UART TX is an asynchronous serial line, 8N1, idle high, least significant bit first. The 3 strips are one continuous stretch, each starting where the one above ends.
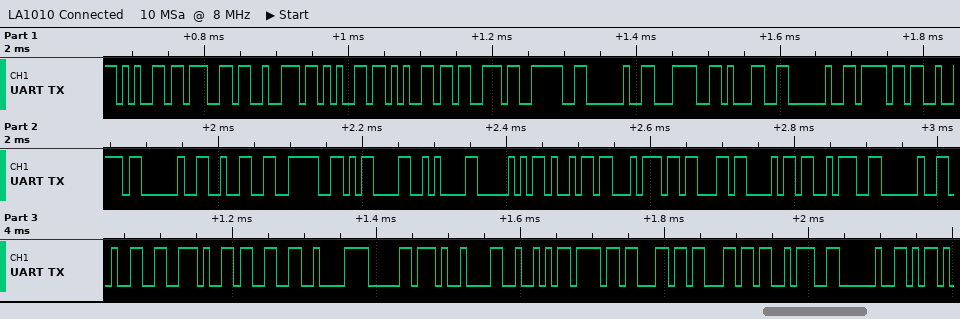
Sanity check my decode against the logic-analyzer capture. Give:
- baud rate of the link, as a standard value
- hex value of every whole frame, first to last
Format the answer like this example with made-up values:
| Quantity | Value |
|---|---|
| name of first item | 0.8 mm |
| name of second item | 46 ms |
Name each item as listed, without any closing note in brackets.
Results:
| Quantity | Value |
|---|---|
| baud rate of the link, as a standard value | 115200 baud |
| hex value of every whole frame, first to last | 65 67 72 65 65 73 3E 20 3C 31 20 6F 72 20 32 3E 0D 0A 50 69 74 63 68 3A 20 32 2E 33 C2 B0 09 52 6F 6C 6C 3A 20 |
